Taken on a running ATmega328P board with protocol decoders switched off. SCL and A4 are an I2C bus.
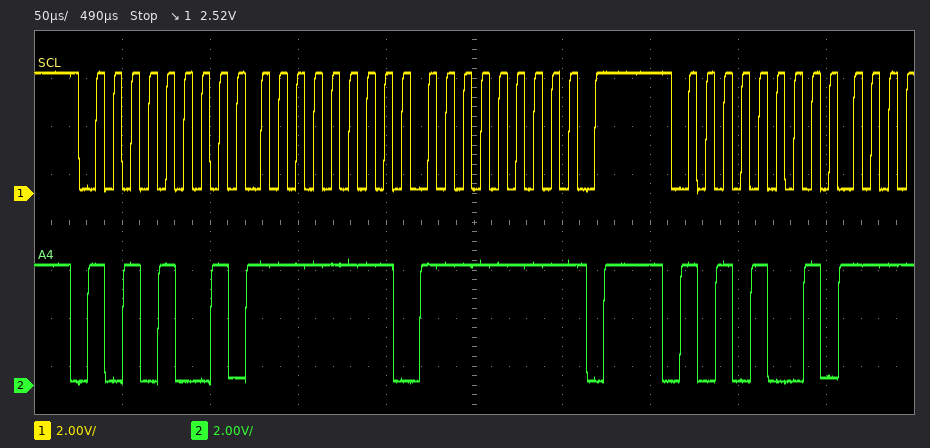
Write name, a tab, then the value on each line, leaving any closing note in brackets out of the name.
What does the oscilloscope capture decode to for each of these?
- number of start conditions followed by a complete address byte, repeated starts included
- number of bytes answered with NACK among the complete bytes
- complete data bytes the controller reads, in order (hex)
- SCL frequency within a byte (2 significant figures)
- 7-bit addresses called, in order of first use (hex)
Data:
number of start conditions followed by a complete address byte, repeated starts included	2
number of bytes answered with NACK among the complete bytes	1
complete data bytes the controller reads, in order	FF FF
SCL frequency within a byte	100 kHz
7-bit addresses called, in order of first use	0x54
